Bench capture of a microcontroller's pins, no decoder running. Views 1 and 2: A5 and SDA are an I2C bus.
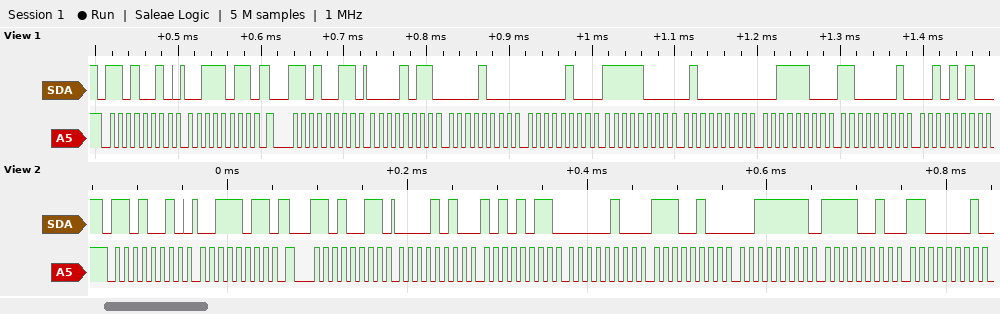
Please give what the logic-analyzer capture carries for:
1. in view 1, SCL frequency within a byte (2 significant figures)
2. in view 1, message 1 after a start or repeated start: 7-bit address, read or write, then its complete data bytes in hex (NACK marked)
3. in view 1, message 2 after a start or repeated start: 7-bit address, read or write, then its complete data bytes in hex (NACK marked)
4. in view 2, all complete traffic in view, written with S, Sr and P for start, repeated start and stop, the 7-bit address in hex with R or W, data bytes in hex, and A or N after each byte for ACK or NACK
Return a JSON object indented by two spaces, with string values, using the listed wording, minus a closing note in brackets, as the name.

{
  "in view 1, SCL frequency within a byte": "100 kHz",
  "in view 1, message 1 after a start or repeated start: 7-bit address, read or write, then its complete data bytes in hex": "0x69 write: 3B",
  "in view 1, message 2 after a start or repeated start: 7-bit address, read or write, then its complete data bytes in hex": "0x69 read: 0B 08 04 F8 40 3C C1 2A",
  "in view 2, all complete traffic in view, written with S, Sr and P for start, repeated start and stop, the 7-bit address in hex with R or W, data bytes in hex, and A or N after each byte for ACK or NACK": "S 69W A 3B A Sr 69R A 0A A AB A 04 A E4 A 3F A F2 A C1 A"
}
